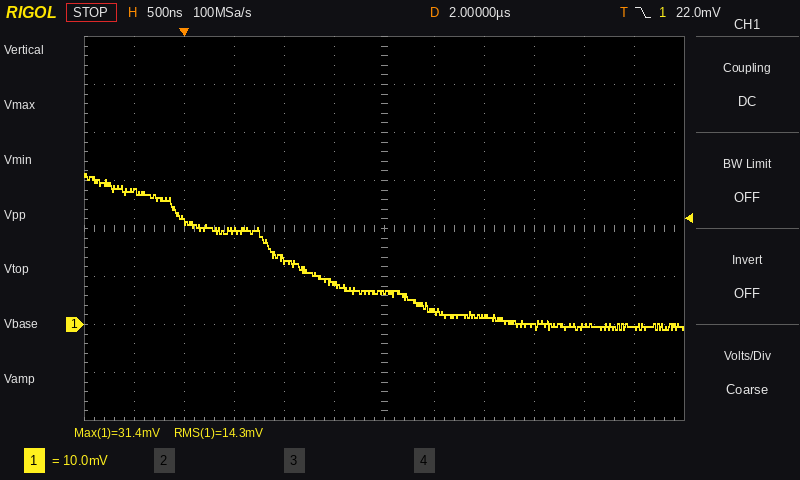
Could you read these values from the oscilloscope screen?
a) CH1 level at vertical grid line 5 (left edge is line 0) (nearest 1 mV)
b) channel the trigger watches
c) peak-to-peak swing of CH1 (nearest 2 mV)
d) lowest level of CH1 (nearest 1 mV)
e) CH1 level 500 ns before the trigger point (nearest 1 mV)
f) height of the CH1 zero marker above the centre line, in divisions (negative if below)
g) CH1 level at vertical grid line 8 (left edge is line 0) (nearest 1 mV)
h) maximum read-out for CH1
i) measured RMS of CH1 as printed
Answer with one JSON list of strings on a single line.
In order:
["8 mV", "CH1", "32 mV", "-1 mV", "28 mV", "-2.0 div", "2 mV", "31.4 mV", "14.3 mV"]
